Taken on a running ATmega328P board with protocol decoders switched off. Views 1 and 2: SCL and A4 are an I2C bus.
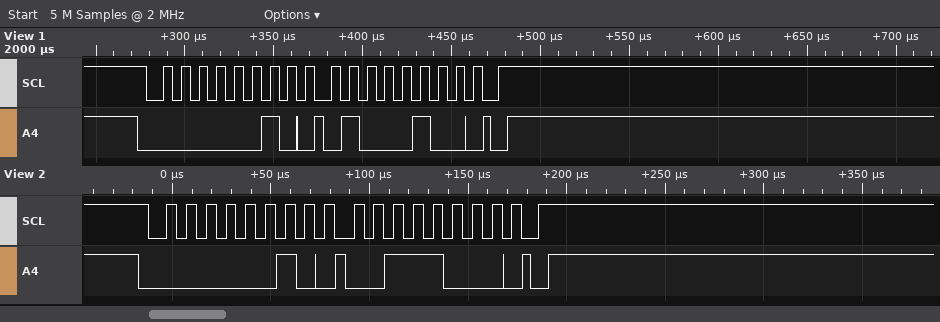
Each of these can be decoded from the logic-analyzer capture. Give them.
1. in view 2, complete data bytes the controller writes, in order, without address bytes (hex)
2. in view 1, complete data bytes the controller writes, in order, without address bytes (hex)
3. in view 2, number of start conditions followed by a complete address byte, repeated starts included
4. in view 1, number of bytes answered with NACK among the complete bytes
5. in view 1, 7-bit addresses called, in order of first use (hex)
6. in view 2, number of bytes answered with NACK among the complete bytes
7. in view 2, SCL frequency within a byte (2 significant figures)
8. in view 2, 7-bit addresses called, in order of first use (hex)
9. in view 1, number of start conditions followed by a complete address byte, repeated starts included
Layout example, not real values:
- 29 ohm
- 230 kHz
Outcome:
- 38
- 44
- 1
- 0
- 0x01
- 0
- 100 kHz
- 0x01
- 1
